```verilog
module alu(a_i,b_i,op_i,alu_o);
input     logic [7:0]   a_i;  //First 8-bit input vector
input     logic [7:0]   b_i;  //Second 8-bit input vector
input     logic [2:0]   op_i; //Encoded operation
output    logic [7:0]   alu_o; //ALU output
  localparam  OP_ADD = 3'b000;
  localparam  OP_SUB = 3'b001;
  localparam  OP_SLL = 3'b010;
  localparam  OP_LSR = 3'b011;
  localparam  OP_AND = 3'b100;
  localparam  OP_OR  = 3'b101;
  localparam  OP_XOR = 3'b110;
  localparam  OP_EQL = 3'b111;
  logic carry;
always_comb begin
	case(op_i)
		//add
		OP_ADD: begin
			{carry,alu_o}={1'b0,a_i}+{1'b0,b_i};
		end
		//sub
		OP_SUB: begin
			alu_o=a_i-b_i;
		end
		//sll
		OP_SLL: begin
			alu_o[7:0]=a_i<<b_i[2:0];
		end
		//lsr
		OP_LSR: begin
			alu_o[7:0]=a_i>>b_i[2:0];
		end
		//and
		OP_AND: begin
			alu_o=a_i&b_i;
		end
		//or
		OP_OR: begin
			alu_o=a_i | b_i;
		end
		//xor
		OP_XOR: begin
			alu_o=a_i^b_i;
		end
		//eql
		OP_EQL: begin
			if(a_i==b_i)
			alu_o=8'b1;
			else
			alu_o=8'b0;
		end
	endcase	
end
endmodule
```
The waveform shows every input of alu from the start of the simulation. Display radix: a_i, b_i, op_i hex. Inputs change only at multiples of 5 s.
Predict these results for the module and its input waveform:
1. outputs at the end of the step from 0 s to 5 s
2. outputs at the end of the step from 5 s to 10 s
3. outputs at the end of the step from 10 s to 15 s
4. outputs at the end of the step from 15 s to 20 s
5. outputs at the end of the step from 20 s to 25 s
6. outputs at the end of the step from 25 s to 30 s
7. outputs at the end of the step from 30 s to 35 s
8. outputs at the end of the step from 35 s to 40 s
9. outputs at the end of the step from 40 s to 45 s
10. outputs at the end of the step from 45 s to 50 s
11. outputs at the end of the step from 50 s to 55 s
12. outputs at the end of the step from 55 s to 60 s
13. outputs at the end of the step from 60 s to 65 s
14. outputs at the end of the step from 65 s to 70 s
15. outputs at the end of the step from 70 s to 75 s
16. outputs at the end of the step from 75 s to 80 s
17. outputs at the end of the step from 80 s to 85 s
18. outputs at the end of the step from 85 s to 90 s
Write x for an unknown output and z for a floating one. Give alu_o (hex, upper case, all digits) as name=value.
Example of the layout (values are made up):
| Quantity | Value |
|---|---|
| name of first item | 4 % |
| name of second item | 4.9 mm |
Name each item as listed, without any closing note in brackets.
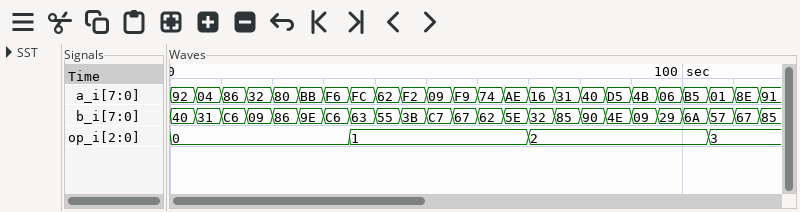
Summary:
| Quantity | Value |
|---|---|
| outputs at the end of the step from 0 s to 5 s | alu_o=D2 |
| outputs at the end of the step from 5 s to 10 s | alu_o=35 |
| outputs at the end of the step from 10 s to 15 s | alu_o=4C |
| outputs at the end of the step from 15 s to 20 s | alu_o=3B |
| outputs at the end of the step from 20 s to 25 s | alu_o=06 |
| outputs at the end of the step from 25 s to 30 s | alu_o=59 |
| outputs at the end of the step from 30 s to 35 s | alu_o=BC |
| outputs at the end of the step from 35 s to 40 s | alu_o=99 |
| outputs at the end of the step from 40 s to 45 s | alu_o=0D |
| outputs at the end of the step from 45 s to 50 s | alu_o=B7 |
| outputs at the end of the step from 50 s to 55 s | alu_o=42 |
| outputs at the end of the step from 55 s to 60 s | alu_o=92 |
| outputs at the end of the step from 60 s to 65 s | alu_o=12 |
| outputs at the end of the step from 65 s to 70 s | alu_o=50 |
| outputs at the end of the step from 70 s to 75 s | alu_o=58 |
| outputs at the end of the step from 75 s to 80 s | alu_o=20 |
| outputs at the end of the step from 80 s to 85 s | alu_o=40 |
| outputs at the end of the step from 85 s to 90 s | alu_o=40 |
